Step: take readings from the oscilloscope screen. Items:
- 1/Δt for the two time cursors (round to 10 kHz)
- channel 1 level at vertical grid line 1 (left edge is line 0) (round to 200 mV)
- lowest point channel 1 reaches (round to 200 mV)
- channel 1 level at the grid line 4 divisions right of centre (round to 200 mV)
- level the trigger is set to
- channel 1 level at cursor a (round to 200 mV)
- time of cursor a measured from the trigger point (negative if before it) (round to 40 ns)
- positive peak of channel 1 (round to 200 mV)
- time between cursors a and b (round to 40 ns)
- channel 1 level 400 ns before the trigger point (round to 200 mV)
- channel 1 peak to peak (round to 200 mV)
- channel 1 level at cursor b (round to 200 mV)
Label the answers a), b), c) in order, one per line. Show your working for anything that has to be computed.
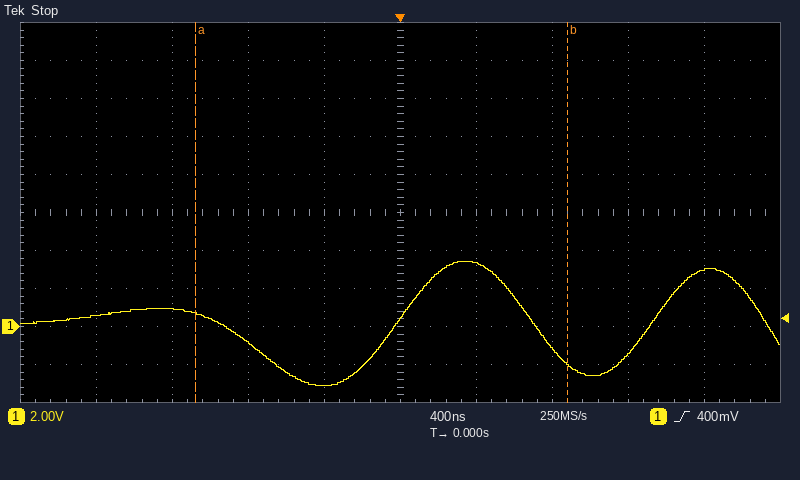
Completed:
a) 1 / 1.96 µs ≈ 510 kHz
b) 600 mV
c) -3.2 V
d) 3.0 V
e) 400 mV
f) 600 mV
g) -1.08 µs
h) 3.4 V
i) 1.96 µs
j) -3.2 V
k) 3.4 V − (-3.2 V) = 6.6 V
l) -2.0 V
